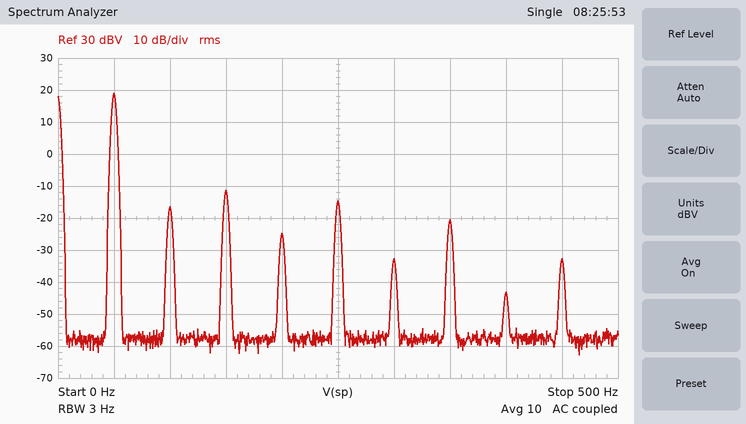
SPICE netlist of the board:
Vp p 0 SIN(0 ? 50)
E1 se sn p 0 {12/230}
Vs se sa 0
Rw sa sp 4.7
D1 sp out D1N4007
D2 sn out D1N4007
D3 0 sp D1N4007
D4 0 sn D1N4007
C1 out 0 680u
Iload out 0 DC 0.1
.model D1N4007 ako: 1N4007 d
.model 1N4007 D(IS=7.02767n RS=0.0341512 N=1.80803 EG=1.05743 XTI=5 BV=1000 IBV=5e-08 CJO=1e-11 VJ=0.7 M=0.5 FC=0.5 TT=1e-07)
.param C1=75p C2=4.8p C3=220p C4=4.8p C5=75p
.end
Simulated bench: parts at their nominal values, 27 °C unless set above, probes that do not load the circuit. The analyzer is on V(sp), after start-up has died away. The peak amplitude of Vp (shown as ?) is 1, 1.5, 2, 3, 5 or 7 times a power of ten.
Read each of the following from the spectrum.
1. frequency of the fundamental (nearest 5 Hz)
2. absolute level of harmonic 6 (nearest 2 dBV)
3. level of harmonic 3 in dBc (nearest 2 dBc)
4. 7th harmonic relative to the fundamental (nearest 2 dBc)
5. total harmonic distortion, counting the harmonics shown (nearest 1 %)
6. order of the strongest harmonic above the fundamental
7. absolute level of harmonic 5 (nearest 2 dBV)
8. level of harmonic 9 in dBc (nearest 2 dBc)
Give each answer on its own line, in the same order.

50 Hz
-32 dBV
-30 dBc
-40 dBc
4 %
3
-14 dBV
-52 dBc
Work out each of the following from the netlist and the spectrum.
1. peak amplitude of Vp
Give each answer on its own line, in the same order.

500 V
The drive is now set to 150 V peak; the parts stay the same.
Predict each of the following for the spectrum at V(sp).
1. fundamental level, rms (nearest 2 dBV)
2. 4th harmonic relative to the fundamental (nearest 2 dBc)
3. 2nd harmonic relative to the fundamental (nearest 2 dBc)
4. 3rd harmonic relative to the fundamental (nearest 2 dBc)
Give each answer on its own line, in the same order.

8 dBV
-38 dBc
-26 dBc
-22 dBc
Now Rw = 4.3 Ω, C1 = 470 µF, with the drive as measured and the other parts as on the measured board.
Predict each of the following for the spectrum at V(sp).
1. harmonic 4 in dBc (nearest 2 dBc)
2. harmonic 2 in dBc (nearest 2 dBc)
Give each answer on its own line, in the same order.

-40 dBc
-32 dBc
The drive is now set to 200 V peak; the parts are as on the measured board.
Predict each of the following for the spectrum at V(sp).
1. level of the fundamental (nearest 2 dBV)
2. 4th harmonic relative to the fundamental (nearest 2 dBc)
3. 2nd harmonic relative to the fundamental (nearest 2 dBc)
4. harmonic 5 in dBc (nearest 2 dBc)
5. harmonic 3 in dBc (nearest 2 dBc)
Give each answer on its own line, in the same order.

10 dBV
-38 dBc
-28 dBc
-30 dBc
-24 dBc
